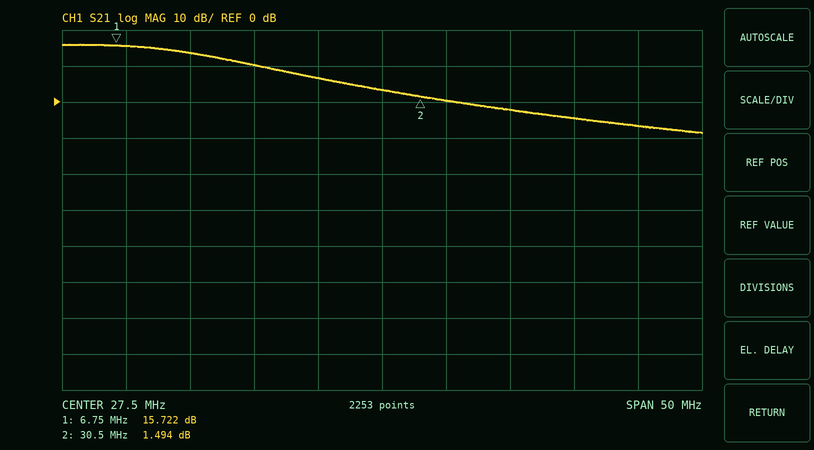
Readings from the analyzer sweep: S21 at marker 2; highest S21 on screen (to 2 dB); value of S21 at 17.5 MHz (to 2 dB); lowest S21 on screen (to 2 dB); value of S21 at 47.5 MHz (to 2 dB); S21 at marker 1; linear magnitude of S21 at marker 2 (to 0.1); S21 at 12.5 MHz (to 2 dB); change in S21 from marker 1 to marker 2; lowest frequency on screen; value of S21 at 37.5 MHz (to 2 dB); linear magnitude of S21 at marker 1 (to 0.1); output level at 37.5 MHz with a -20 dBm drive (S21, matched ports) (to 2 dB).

1.494 dB
16 dB
10 dB
-8 dB
-6 dB
15.722 dB
1.2
14 dB
-14.228 dB
2.5 MHz
-2 dB
6.1
-22 dBm
